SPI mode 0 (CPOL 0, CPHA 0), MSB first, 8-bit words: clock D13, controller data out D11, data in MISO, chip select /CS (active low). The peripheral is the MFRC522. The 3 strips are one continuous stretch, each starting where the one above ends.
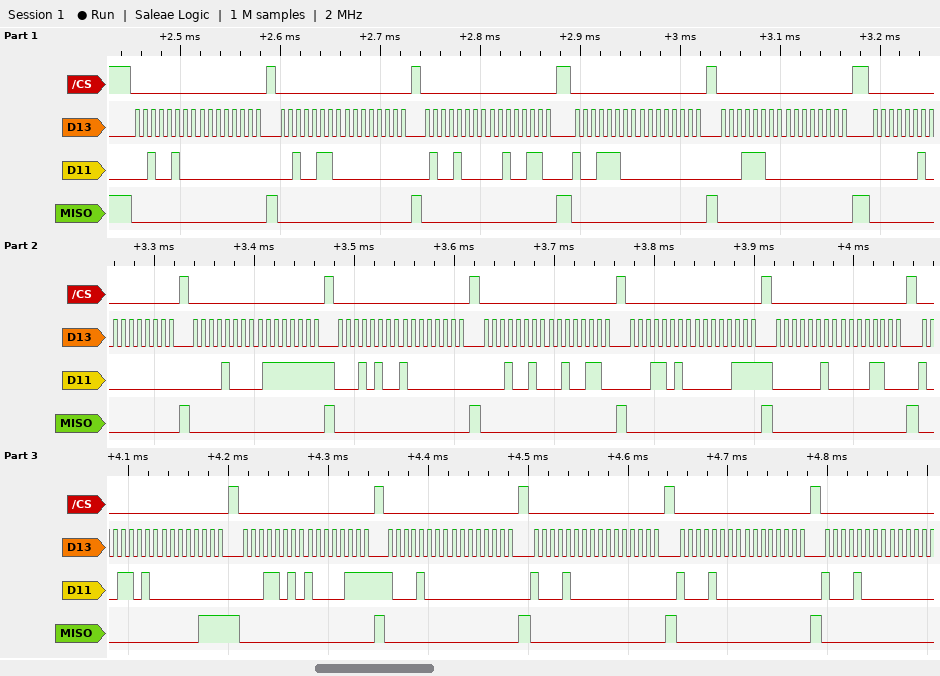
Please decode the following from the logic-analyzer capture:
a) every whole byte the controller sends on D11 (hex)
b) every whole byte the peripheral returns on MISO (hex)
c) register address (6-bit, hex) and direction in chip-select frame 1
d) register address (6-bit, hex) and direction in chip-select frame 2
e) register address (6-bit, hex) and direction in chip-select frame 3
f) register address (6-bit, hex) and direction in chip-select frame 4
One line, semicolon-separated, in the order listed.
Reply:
24 00 26 00 48 26 9C 00 1C 00 02 00 08 7F 14 80 12 26 1A 07 02 0C 9A 00 1A 87 88 00 88 00 88 00 88; 00 00 00 00 00 00 00 00 00 00 00 00 00 00 00 00 00 00 00 00 00 00 00 07 00 00 00 00 00 00 00 00 00; 0x12 write; 0x13 write; 0x24 write; 0x0E read
